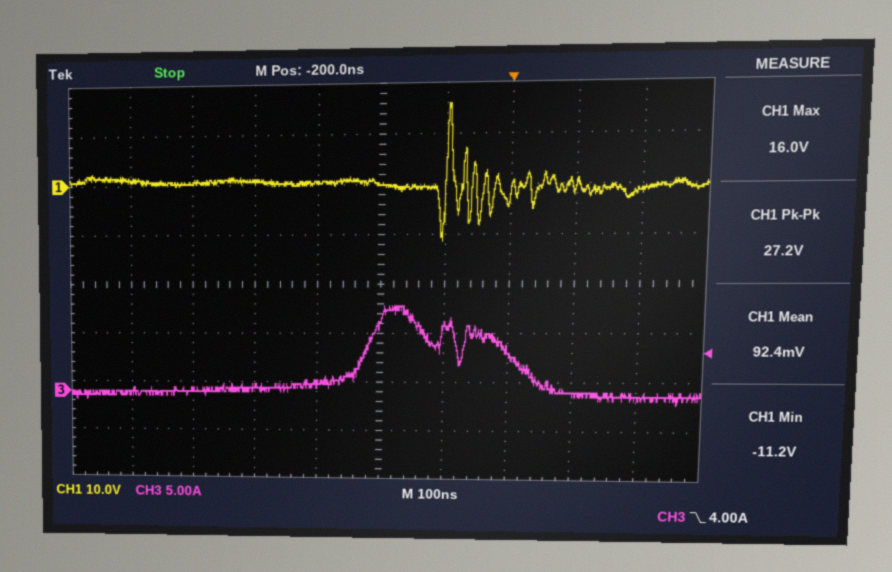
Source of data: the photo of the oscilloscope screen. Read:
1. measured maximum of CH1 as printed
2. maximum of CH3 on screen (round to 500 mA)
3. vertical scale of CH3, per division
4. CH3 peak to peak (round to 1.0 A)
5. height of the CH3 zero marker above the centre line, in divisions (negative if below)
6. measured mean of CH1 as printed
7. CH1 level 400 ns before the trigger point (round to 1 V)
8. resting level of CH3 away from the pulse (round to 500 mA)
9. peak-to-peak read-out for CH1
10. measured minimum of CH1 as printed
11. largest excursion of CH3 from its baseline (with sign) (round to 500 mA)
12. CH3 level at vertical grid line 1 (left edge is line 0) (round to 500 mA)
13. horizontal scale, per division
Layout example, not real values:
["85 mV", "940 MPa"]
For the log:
["16.0 V", "9.0 A", "5 A", "10.0 A", "-2.2 div", "92.4 mV", "1 V", "0.0 A", "27.2 V", "-11.2 V", "+9.0 A", "0.0 A", "100 ns"]
